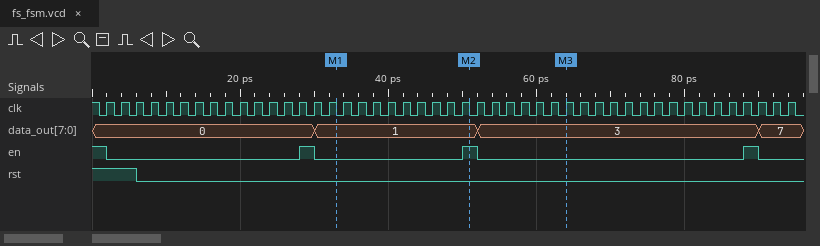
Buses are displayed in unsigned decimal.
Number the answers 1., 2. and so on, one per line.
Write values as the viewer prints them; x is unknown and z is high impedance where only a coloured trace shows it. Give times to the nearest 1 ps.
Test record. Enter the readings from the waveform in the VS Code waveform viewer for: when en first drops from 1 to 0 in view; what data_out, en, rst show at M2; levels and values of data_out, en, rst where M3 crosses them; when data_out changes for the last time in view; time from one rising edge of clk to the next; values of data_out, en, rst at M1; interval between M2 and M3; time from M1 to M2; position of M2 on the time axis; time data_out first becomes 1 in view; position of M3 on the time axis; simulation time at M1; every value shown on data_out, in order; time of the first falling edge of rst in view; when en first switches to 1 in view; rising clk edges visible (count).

1. 2 ps
2. data_out=1, en=1, rst=0
3. data_out=3, en=0, rst=0
4. 90 ps
5. 2 ps
6. data_out=1, en=0, rst=0
7. 13 ps
8. 18 ps
9. 51 ps
10. 30 ps
11. 64 ps
12. 33 ps
13. 0, 1, 3, 7
14. 6 ps
15. 28 ps
16. 47
